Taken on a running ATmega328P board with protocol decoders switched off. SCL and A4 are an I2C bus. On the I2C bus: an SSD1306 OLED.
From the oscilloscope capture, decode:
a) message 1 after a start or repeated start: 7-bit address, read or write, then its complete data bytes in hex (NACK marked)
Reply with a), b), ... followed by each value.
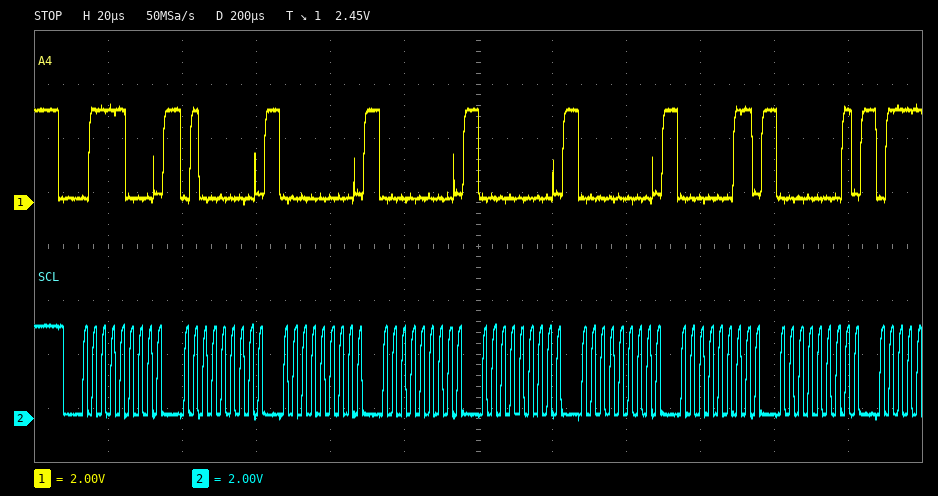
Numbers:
a) 0x3C write: 40 00 00 00 00 03 01
